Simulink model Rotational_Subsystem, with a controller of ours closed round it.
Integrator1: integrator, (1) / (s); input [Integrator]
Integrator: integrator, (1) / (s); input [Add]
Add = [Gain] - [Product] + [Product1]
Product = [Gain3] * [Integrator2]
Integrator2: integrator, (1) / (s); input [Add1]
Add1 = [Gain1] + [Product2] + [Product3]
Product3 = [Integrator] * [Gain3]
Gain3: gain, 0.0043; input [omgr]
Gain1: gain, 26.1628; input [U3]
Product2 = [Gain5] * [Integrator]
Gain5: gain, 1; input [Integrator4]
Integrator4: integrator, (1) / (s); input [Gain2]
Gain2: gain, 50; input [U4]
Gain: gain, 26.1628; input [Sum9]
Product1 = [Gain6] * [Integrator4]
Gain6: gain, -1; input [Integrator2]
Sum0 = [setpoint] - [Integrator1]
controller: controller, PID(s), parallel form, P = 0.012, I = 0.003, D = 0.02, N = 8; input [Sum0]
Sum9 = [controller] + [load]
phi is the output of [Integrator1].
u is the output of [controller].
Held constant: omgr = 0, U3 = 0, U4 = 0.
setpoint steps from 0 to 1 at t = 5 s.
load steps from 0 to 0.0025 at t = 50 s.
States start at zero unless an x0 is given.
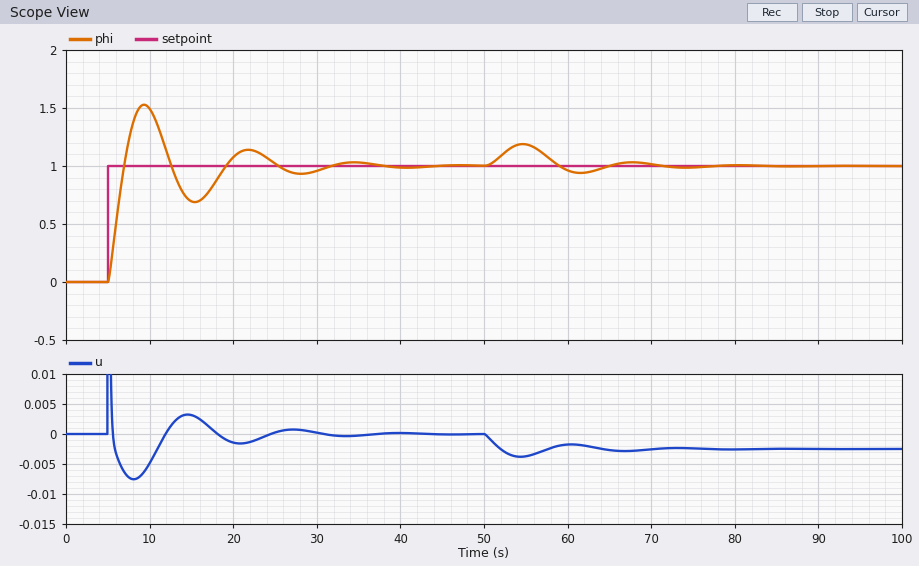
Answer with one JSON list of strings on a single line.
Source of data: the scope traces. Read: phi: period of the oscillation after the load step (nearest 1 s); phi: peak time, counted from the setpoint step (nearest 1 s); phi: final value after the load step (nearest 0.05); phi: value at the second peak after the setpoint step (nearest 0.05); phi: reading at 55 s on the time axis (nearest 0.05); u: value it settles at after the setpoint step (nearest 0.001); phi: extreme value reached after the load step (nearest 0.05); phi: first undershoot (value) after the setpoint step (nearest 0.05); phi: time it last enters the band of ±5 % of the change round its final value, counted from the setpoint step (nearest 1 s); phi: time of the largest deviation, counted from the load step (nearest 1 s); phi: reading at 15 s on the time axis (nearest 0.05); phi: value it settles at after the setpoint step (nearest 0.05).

["13 s", "4 s", "1.00", "1.15", "1.20", "0.000", "1.20", "0.70", "25 s", "5 s", "0.70", "1.00"]
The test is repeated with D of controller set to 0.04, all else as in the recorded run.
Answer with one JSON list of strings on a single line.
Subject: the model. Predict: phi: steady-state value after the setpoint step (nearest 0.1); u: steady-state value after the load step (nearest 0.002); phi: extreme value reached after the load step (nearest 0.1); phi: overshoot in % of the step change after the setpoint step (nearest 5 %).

["1.0", "-0.002", "1.1", "25 %"]
